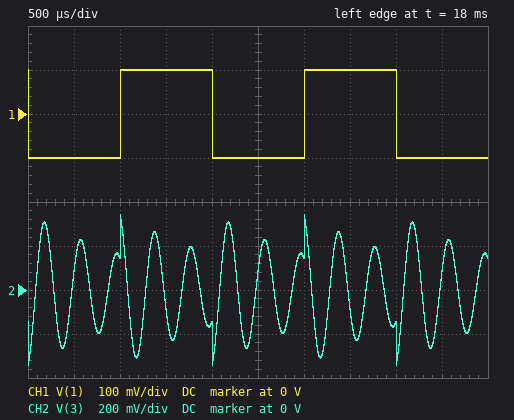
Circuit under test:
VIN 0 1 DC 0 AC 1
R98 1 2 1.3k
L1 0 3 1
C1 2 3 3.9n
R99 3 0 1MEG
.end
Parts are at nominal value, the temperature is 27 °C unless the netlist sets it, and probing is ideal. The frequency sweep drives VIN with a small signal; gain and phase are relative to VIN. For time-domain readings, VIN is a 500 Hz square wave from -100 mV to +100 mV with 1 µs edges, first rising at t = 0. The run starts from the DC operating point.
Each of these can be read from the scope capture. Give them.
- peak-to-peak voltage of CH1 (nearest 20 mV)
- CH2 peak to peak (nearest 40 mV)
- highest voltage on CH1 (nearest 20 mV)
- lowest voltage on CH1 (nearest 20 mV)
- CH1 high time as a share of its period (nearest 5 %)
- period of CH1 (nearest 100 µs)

200 mV
680 mV
100 mV
-100 mV
50 %
2.0 ms
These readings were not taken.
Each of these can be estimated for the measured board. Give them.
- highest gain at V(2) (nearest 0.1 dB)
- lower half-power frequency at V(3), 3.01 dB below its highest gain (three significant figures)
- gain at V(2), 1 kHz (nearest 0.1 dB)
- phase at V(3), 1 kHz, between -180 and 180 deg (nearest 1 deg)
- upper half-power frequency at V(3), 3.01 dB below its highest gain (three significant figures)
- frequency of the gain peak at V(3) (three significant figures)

0 dB
2.44 kHz
0 dB
-3 deg
2.69 kHz
2.55 kHz
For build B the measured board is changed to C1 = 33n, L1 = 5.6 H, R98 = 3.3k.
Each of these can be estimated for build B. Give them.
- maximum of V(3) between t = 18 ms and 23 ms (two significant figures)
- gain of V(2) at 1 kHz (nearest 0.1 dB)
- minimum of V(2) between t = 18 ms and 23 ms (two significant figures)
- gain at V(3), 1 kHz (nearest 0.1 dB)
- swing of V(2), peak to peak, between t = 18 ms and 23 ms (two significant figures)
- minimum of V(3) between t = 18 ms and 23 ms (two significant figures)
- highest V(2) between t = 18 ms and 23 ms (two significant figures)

250 mV
-0.1 dB
-150 mV
1.2 dB
300 mV
-250 mV
150 mV
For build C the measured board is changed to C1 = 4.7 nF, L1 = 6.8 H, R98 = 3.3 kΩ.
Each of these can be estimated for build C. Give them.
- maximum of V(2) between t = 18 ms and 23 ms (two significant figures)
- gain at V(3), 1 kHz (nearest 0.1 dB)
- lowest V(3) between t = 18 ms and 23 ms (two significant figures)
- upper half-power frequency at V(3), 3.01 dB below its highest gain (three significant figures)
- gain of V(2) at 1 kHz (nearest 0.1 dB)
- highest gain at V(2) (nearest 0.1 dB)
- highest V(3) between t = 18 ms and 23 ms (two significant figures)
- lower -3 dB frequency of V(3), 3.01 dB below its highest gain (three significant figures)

110 mV
12.5 dB
-120 mV
954 Hz
-1.1 dB
0 dB
120 mV
841 Hz
